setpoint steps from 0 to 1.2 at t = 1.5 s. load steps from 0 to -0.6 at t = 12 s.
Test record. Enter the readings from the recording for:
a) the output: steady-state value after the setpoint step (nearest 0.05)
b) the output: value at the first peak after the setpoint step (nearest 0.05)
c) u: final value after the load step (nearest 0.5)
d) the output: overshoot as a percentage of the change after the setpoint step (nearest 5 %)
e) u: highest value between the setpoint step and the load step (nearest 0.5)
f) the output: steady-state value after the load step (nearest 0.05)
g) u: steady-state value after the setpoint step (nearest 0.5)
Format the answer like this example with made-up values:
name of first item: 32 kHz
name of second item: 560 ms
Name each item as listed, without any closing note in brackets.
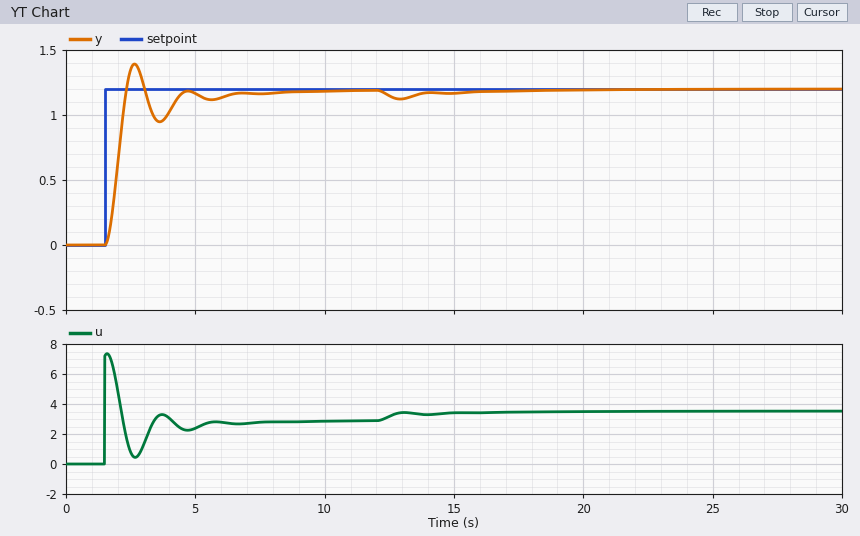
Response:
the output: steady-state value after the setpoint step: 1.20
the output: value at the first peak after the setpoint step: 1.40
u: final value after the load step: 3.5
the output: overshoot as a percentage of the change after the setpoint step: 15 %
u: highest value between the setpoint step and the load step: 7.5
the output: steady-state value after the load step: 1.20
u: steady-state value after the setpoint step: 3.0
